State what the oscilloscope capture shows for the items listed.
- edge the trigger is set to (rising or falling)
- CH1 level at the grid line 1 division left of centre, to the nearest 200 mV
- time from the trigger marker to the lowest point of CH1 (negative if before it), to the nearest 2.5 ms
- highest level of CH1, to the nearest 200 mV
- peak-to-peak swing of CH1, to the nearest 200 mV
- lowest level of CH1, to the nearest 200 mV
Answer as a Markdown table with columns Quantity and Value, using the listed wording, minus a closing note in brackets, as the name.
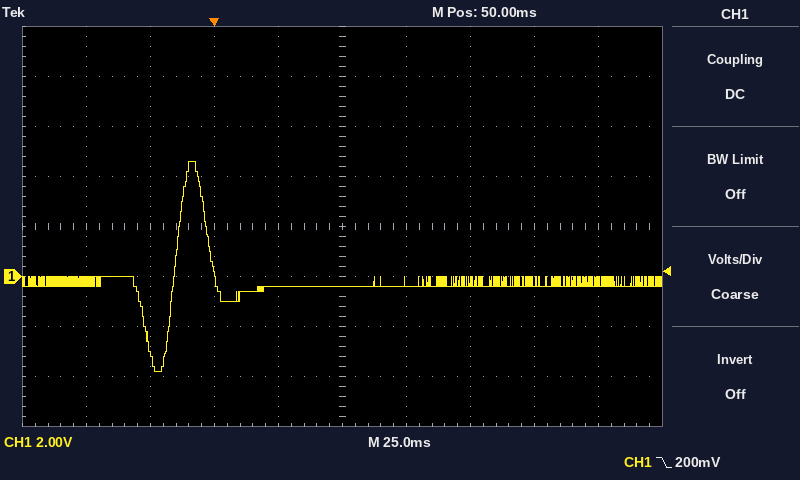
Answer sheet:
| Quantity | Value |
|---|---|
| edge the trigger is set to | falling |
| CH1 level at the grid line 1 division left of centre, to the nearest 200 mV | -400 mV |
| time from the trigger marker to the lowest point of CH1 (negative if before it), to the nearest 2.5 ms | -22.5 ms |
| highest level of CH1, to the nearest 200 mV | 4.6 V |
| peak-to-peak swing of CH1, to the nearest 200 mV | 8.4 V |
| lowest level of CH1, to the nearest 200 mV | -3.8 V |
